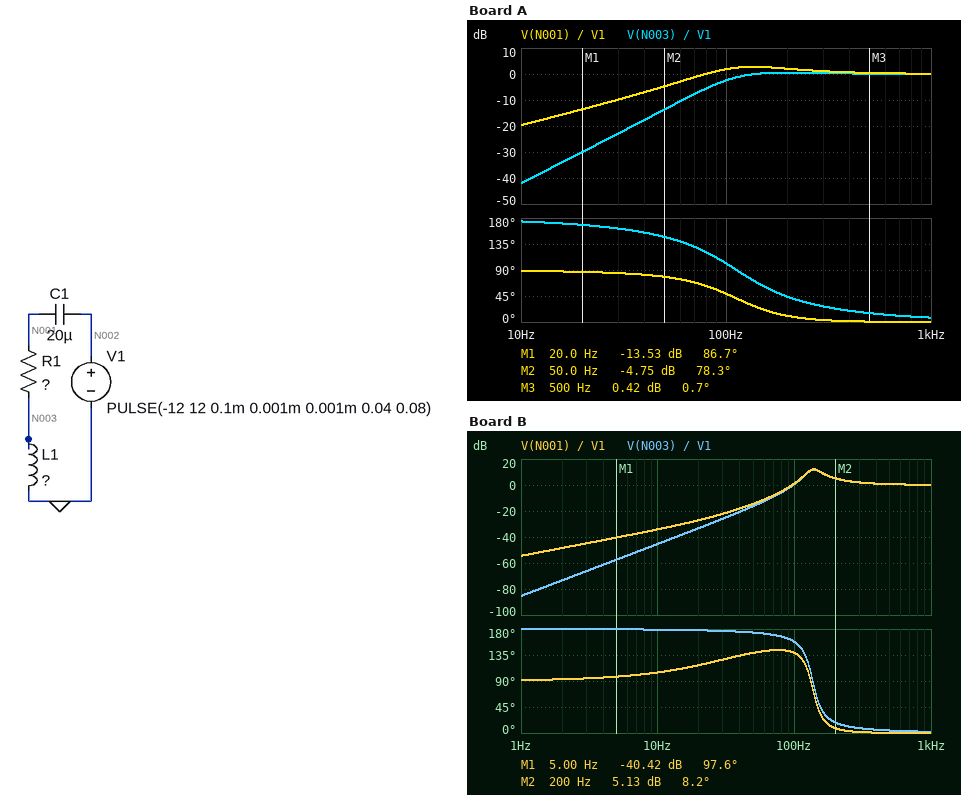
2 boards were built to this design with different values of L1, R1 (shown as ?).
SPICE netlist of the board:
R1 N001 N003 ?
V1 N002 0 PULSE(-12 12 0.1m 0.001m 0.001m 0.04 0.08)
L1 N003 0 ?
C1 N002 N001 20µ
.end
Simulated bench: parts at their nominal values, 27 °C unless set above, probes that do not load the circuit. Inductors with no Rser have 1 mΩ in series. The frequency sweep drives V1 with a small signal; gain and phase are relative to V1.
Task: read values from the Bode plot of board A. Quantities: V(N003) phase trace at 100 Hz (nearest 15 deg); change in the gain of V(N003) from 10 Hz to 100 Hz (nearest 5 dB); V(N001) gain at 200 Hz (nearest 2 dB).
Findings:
105 deg
40 dB
2 dB
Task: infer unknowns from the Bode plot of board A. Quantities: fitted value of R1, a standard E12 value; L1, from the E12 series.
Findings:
82 Ω
100 mH
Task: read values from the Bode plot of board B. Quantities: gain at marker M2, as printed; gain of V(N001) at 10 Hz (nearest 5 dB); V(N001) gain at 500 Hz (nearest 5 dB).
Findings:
5.13 dB
-35 dB
0 dB
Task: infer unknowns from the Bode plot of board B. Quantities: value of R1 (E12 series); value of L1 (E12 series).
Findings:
15 Ω
68 mH
